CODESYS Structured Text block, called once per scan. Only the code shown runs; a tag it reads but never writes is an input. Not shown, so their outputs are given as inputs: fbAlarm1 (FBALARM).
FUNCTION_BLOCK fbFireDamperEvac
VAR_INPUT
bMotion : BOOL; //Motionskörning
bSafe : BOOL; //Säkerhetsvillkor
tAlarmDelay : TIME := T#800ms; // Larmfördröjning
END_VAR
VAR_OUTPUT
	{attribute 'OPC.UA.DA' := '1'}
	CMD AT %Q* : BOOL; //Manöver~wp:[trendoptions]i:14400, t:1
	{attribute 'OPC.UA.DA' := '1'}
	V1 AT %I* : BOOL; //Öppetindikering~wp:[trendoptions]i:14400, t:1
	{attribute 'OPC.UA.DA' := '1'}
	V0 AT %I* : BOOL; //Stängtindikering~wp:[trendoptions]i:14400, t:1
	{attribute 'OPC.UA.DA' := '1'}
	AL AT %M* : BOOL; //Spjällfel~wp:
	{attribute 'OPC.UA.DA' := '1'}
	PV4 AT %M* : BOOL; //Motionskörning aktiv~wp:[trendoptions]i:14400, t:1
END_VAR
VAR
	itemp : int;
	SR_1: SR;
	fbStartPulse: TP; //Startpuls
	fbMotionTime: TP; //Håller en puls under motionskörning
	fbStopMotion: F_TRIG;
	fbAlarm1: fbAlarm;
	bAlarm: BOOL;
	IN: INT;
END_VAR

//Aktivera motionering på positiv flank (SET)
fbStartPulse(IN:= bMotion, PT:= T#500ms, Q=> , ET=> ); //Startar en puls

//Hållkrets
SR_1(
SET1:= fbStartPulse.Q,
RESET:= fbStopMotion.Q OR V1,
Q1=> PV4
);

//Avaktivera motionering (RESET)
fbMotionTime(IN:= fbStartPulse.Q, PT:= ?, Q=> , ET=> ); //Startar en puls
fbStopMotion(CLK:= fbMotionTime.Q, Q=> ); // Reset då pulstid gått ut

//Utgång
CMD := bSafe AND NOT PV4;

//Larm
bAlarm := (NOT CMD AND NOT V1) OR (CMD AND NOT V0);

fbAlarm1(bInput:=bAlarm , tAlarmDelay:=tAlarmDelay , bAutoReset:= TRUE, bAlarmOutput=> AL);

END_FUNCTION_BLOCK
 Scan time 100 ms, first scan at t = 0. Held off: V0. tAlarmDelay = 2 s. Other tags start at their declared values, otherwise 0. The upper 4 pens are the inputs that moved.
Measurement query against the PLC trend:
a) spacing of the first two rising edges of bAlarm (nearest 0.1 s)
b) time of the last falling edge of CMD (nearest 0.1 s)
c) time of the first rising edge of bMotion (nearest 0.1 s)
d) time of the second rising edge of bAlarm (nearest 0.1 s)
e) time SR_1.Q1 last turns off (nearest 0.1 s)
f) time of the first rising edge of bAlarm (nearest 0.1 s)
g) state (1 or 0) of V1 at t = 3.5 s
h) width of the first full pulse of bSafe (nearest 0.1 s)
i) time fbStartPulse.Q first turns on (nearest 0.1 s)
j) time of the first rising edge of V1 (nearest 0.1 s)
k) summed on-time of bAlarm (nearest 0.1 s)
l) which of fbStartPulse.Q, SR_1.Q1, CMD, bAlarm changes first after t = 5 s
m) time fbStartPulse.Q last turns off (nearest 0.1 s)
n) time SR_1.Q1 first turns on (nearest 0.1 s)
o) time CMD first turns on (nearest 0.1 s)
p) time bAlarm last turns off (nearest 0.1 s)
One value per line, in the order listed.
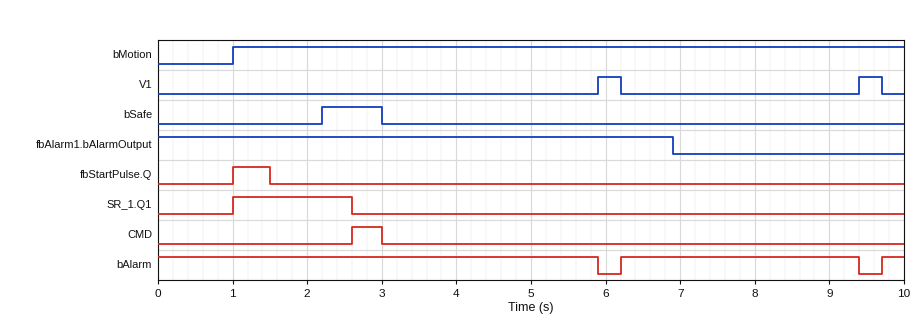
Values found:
3.5 s
3.0 s
1.0 s
9.7 s
2.6 s
6.2 s
0
0.8 s
1.0 s
5.9 s
9.4 s
bAlarm
1.5 s
1.0 s
2.6 s
9.4 s
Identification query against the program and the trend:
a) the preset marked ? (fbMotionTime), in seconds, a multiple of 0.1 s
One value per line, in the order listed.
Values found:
1.5 s
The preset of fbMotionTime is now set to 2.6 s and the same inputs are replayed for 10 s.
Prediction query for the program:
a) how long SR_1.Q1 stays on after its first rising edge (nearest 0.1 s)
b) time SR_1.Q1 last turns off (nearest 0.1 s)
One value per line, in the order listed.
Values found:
2.7 s
3.7 s
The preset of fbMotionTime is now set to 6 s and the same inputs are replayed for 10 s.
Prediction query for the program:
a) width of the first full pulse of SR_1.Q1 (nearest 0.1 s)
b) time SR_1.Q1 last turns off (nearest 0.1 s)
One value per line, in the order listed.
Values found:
4.9 s
5.9 s
